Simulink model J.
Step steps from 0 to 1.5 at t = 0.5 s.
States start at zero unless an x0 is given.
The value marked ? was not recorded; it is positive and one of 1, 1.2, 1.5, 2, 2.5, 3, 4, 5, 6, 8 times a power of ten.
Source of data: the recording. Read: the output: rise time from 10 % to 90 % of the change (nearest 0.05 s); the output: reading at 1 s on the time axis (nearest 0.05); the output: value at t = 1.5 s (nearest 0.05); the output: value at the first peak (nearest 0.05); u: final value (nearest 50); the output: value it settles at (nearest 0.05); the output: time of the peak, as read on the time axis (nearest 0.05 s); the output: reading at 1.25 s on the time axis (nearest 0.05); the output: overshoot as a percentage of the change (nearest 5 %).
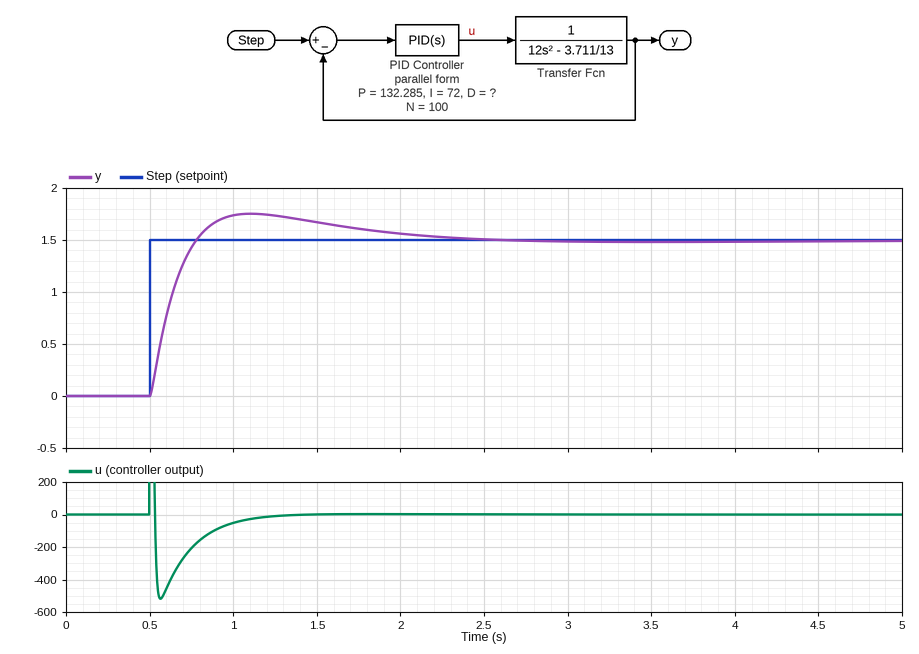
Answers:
0.20 s
1.75
1.65
1.75
0
1.50
1.10 s
1.75
15 %
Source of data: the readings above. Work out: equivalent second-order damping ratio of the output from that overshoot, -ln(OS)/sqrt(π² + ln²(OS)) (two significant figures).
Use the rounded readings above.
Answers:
0.52
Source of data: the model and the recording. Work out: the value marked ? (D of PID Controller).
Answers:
80
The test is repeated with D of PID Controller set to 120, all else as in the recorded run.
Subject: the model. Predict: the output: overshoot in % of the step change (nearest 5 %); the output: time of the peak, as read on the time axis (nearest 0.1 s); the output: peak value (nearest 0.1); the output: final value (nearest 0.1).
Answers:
10 %
1.0 s
1.6
1.5
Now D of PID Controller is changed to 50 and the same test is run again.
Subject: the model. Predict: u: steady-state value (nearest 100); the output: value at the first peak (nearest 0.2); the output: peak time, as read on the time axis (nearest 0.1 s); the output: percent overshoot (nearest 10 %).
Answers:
0
2.0
1.2 s
30 %
